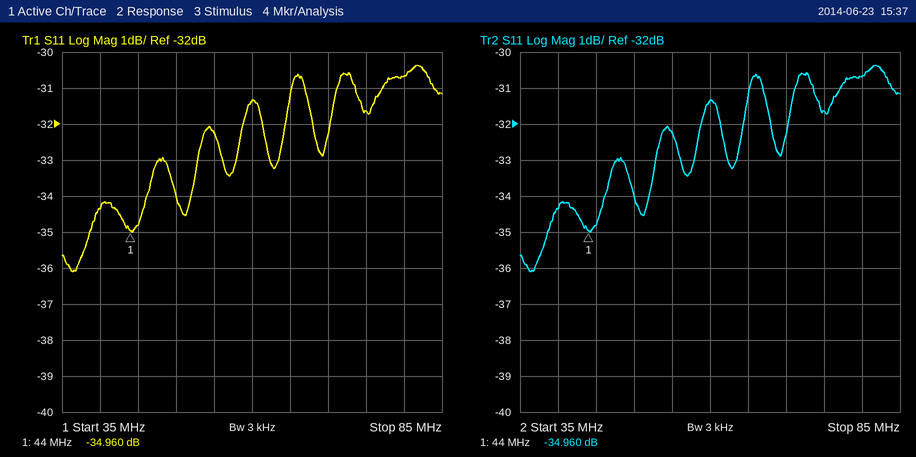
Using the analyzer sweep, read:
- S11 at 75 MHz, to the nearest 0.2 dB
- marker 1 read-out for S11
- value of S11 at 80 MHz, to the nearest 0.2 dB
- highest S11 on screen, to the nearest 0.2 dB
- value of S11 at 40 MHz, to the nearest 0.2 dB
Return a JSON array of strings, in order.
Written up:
["-31.6 dB", "-34.960 dB", "-30.6 dB", "-30.4 dB", "-34.4 dB"]
